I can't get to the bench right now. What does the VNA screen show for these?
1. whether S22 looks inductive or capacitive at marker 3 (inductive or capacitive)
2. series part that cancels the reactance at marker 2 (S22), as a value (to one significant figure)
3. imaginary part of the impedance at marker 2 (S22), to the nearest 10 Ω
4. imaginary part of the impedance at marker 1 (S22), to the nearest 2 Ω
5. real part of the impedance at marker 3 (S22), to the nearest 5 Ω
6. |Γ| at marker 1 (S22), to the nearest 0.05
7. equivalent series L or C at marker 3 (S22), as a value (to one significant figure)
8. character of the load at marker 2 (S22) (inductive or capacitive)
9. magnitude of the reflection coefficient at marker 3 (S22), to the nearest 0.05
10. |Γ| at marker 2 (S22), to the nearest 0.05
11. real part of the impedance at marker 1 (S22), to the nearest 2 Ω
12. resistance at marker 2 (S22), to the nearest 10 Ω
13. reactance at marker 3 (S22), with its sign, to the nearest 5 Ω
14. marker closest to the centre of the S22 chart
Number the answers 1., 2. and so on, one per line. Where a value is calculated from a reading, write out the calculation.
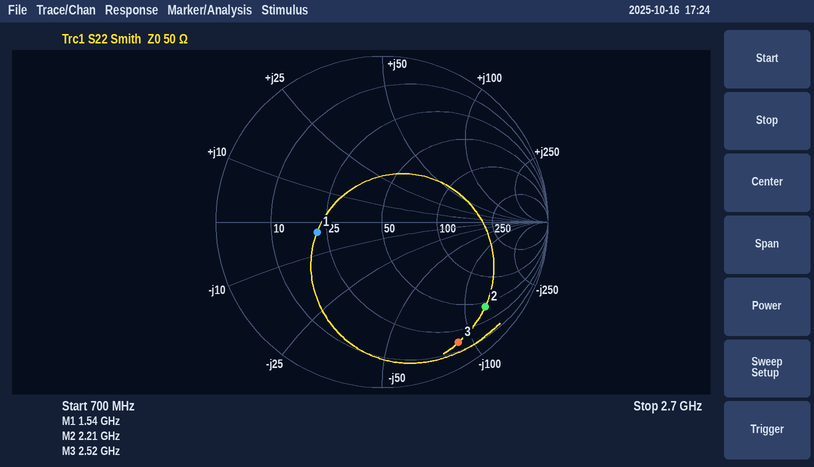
1. capacitive
2. L = 130 Ω/(2π × 2.21 GHz) ≈ 9 nH
3. -130 Ω
4. -4 Ω
5. 15 Ω
6. 0.40
7. C = 1/(2π × 2.52 GHz × 90 Ω) ≈ 702 fF, so 700 fF to one significant figure
8. capacitive
9. 0.85
10. 0.80
11. 22 Ω
12. 40 Ω
13. -90 Ω
14. marker 1
